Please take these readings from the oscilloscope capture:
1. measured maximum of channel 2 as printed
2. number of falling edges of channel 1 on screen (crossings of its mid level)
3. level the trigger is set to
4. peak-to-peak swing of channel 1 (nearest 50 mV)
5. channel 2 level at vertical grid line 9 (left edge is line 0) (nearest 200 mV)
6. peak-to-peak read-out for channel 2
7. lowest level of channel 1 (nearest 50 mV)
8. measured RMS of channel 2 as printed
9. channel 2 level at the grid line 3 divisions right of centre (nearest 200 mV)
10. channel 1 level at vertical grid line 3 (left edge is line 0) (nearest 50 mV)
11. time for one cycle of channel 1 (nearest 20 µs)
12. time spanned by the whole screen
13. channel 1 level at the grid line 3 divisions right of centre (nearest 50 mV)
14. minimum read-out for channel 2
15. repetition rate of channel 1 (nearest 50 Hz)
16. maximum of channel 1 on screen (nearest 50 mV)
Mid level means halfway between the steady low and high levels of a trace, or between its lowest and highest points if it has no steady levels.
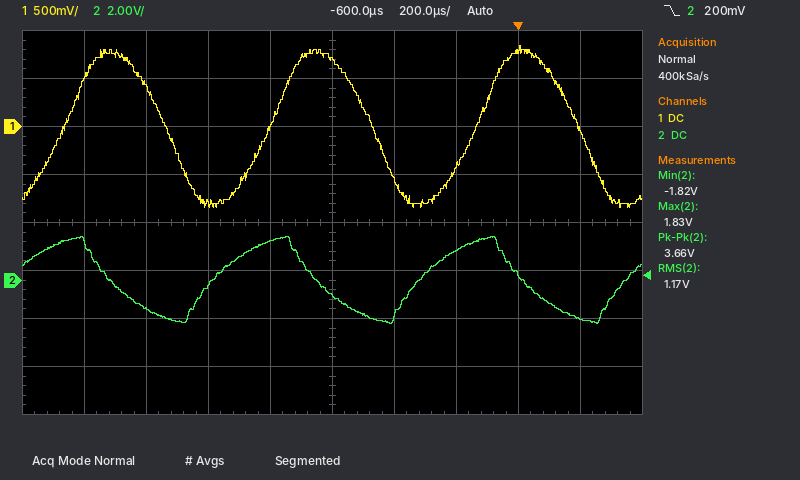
1.83 V
3
200 mV
1.70 V
-1.6 V
3.66 V
-850 mV
1.17 V
200 mV
-800 mV
660 µs
2 ms
800 mV
-1.82 V
1.50 kHz
850 mV
